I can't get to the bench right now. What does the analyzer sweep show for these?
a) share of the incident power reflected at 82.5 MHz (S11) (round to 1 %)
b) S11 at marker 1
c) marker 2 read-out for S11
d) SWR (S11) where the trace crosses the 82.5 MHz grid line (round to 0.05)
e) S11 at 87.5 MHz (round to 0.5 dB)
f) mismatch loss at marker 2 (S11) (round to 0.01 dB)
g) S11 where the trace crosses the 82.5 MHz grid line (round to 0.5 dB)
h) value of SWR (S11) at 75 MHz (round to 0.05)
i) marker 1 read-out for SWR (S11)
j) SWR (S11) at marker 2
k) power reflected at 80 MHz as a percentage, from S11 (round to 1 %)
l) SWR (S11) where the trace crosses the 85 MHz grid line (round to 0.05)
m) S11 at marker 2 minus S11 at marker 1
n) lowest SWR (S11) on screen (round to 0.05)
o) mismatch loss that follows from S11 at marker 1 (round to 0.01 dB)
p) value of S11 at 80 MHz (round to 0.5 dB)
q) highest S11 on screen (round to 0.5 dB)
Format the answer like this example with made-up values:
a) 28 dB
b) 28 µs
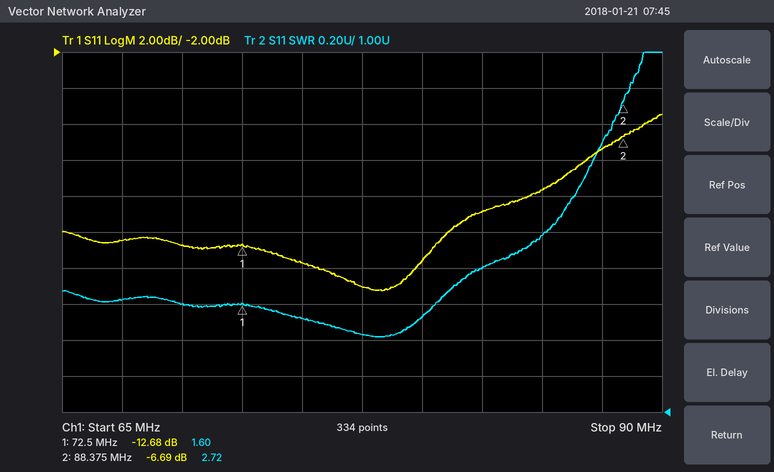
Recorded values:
a) 8 %
b) -12.68 dB
c) -6.69 dB
d) 1.80
e) -7.5 dB
f) 1.05 dB
g) -11.0 dB
h) 1.50
i) 1.60
j) 2.72
k) 4 %
l) 2.00
m) 5.99 dB
n) 1.40
o) 0.24 dB
p) -13.5 dB
q) -5.5 dB
